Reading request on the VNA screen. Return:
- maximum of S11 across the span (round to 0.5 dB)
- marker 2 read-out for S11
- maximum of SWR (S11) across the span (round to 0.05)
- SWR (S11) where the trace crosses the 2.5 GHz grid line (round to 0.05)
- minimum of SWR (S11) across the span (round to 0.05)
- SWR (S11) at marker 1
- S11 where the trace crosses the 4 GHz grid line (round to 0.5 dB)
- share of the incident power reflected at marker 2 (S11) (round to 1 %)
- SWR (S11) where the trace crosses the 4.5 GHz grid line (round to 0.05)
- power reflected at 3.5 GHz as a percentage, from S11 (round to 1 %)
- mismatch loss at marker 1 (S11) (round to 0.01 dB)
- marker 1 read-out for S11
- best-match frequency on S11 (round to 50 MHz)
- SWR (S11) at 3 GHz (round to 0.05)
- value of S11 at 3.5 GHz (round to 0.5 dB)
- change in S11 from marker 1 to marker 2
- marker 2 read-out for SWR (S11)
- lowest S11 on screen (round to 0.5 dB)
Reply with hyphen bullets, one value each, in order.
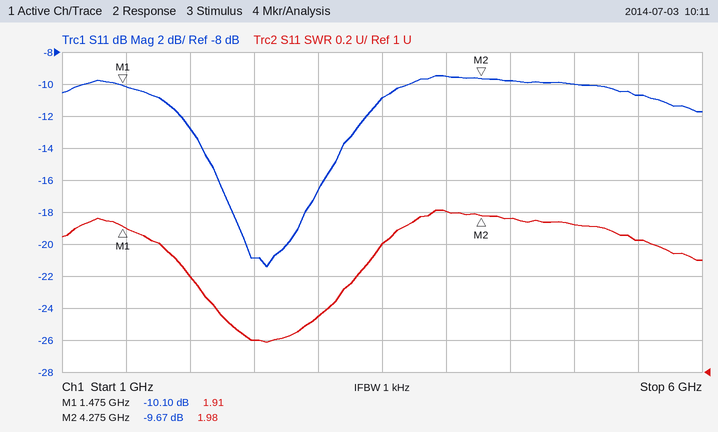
- -9.5 dB
- -9.67 dB
- 2.00
- 1.20
- 1.20
- 1.91
- -9.5 dB
- 11 %
- 1.95
- 8 %
- 0.45 dB
- -10.10 dB
- 2.60 GHz
- 1.35
- -11.0 dB
- 0.43 dB
- 1.98
- -21.5 dB
